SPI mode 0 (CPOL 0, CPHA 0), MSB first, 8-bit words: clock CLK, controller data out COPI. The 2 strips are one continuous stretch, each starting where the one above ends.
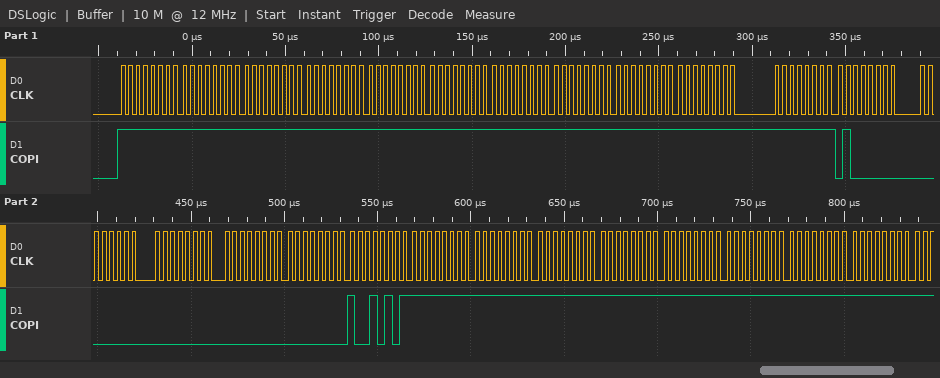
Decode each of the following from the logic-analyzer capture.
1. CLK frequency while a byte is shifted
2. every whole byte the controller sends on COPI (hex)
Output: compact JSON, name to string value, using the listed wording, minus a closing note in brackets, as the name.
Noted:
{"CLK frequency while a byte is shifted": "250 kHz", "every whole byte the controller sends on COPI": "FF FF FF FF FF FF FF FF FF FF FF 40 00 00 00 00 95 FF FF FF FF FF FF FF FF"}
